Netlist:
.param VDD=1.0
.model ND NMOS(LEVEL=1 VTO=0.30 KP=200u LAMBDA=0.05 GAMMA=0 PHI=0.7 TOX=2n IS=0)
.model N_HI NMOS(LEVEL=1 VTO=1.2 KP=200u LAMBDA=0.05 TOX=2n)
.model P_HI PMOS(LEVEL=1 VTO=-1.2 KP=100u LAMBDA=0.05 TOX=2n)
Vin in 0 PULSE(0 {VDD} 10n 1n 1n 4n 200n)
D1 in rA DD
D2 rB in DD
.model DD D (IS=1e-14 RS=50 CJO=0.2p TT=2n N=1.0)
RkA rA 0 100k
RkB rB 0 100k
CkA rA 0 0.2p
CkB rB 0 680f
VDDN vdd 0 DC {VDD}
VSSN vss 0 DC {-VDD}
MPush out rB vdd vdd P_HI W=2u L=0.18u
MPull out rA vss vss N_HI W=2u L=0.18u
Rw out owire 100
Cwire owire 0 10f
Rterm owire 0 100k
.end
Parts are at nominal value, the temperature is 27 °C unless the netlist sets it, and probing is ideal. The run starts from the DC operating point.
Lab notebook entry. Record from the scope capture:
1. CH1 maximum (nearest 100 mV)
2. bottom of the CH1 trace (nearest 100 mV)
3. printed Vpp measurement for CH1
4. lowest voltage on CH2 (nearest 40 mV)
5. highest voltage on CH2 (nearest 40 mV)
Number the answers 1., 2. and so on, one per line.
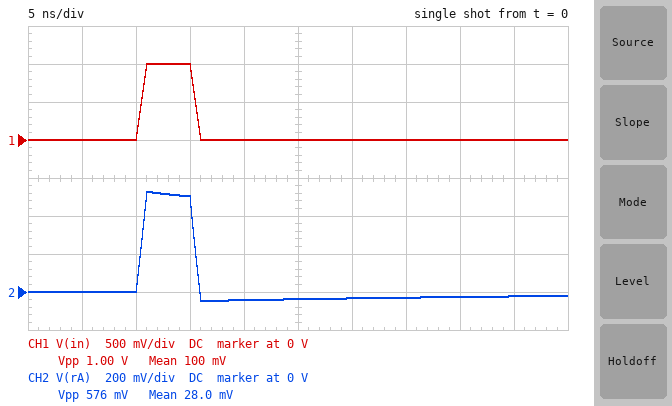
1. 1.0 V
2. 0 V
3. 1.00 V
4. -40 mV
5. 520 mV
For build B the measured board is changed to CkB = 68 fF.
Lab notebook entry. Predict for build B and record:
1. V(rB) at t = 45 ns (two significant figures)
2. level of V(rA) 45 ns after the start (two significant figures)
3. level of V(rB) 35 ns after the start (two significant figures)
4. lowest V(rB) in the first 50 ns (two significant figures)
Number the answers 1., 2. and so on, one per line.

1. -40 mV
2. -23 mV
3. -59 mV
4. -120 mV
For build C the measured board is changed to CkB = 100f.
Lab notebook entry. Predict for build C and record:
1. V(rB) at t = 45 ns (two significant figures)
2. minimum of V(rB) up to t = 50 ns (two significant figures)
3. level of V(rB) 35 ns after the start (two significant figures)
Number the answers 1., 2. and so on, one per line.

1. -36 mV
2. -96 mV
3. -51 mV
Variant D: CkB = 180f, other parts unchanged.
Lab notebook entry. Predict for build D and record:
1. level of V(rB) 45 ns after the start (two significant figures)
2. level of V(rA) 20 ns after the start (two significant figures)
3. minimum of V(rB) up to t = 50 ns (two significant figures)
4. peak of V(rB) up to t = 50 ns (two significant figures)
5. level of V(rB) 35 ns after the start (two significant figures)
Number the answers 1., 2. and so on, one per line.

1. -28 mV
2. -43 mV
3. -60 mV
4. 490 mV
5. -36 mV
